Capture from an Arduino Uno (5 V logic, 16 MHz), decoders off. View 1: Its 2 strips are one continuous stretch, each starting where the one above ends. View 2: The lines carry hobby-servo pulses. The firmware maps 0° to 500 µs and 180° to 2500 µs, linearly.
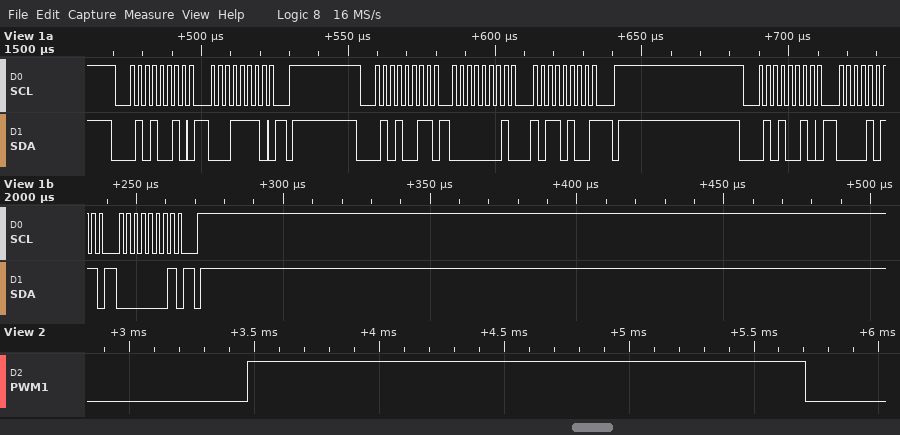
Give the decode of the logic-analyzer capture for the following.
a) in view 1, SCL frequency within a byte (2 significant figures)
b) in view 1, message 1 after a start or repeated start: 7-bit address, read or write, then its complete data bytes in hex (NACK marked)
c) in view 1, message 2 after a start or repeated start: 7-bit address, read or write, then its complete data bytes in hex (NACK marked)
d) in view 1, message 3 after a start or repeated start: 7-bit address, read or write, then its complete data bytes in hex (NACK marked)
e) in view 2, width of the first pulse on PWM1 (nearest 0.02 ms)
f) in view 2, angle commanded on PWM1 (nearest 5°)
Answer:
400 kHz
0x29 write: 1E
0x29 read: 01 B4 NACK
0x29 write: 0B 01
2.24 ms
155°
